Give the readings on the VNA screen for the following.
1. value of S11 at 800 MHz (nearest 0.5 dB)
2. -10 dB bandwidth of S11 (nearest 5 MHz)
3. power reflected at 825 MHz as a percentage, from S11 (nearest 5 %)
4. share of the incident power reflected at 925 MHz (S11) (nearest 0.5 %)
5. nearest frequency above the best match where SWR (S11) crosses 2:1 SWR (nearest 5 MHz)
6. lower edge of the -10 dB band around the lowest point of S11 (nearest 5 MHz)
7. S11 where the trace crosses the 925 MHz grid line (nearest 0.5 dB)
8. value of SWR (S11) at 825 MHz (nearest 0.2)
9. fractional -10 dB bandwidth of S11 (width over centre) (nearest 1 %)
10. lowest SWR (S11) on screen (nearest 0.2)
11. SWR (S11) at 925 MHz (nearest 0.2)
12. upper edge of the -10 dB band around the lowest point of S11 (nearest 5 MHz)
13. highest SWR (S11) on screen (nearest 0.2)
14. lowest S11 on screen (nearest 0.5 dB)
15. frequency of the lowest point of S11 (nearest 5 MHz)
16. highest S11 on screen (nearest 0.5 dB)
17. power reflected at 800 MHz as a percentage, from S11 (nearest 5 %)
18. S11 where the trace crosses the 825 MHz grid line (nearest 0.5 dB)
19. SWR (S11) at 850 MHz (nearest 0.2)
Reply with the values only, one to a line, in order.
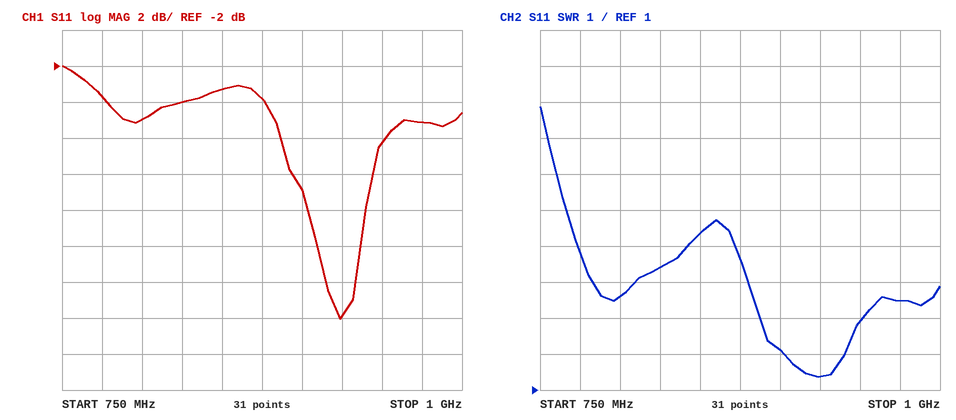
-5.0 dB
35 MHz
40 %
2.5 %
940 MHz
905 MHz
-16.0 dB
4.4
4 %
1.4
1.4
940 MHz
8.8
-16.0 dB
925 MHz
-2.0 dB
30 %
-4.0 dB
5.4
